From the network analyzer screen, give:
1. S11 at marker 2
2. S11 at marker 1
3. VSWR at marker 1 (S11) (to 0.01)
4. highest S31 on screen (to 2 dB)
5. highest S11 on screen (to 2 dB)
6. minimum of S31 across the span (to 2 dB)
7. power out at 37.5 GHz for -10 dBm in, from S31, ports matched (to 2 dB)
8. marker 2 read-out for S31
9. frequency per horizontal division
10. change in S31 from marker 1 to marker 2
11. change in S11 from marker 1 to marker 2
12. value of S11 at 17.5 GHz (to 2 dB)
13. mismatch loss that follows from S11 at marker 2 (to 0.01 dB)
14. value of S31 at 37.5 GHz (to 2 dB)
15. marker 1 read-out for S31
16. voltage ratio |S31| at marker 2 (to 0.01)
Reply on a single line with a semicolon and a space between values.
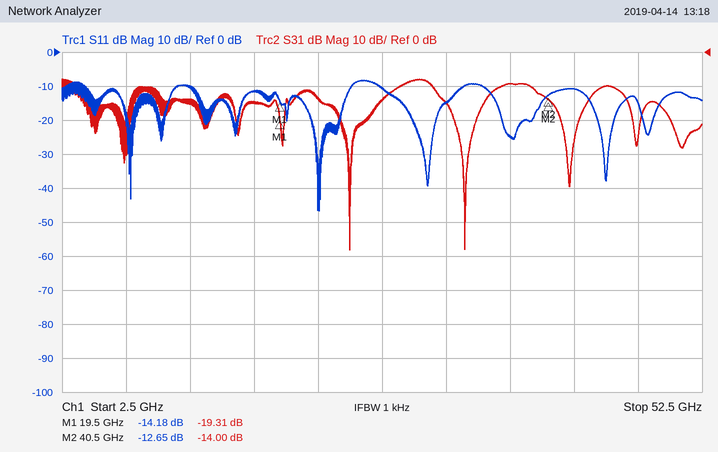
-12.65 dB; -14.18 dB; 1.49; -8 dB; -8 dB; -58 dB; -20 dBm; -14.00 dB; 5 GHz; 5.31 dB; 1.53 dB; -12 dB; 0.24 dB; -10 dB; -19.31 dB; 0.20
